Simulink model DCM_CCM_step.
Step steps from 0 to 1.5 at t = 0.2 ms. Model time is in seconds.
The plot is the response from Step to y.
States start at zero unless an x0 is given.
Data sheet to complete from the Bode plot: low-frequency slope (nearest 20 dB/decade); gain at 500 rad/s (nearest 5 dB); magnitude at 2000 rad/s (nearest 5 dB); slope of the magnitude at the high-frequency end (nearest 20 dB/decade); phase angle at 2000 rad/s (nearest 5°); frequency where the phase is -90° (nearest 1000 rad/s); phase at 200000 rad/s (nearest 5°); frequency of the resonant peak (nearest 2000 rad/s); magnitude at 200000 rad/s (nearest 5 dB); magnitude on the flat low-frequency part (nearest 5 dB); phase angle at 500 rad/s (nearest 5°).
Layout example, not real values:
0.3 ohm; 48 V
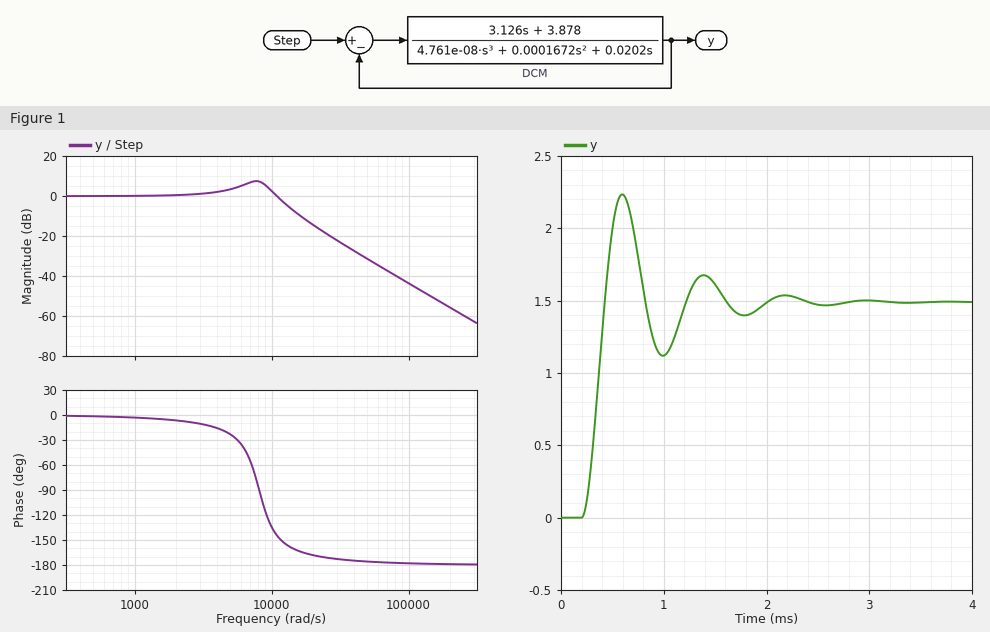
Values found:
0 dB/decade; 0 dB; 0 dB; -40 dB/decade; -5°; 8000 rad/s; -180°; 8000 rad/s; -55 dB; 0 dB; 0°
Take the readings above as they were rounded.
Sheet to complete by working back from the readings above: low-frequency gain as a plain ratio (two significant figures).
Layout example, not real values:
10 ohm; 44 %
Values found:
1.0
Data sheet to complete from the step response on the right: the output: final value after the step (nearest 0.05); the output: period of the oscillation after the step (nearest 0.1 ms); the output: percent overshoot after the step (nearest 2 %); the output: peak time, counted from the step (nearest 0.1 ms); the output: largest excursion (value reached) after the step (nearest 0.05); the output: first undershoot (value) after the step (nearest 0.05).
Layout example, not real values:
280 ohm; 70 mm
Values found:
1.50; 0.8 ms; 50 %; 0.4 ms; 2.25; 1.10
